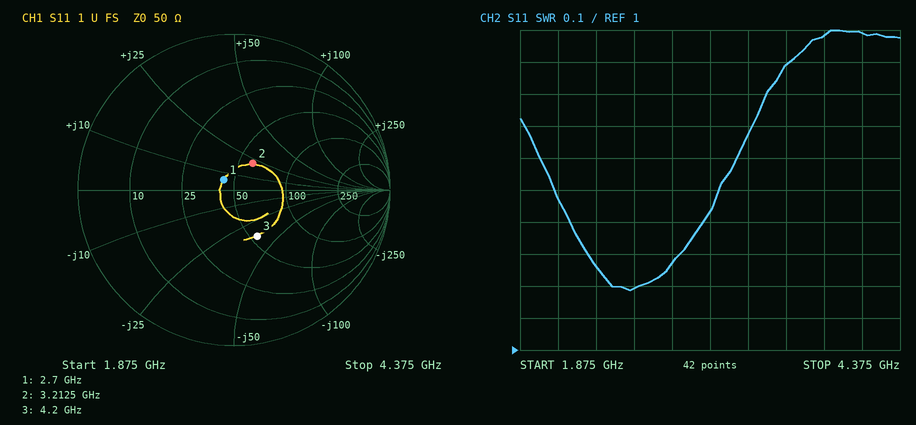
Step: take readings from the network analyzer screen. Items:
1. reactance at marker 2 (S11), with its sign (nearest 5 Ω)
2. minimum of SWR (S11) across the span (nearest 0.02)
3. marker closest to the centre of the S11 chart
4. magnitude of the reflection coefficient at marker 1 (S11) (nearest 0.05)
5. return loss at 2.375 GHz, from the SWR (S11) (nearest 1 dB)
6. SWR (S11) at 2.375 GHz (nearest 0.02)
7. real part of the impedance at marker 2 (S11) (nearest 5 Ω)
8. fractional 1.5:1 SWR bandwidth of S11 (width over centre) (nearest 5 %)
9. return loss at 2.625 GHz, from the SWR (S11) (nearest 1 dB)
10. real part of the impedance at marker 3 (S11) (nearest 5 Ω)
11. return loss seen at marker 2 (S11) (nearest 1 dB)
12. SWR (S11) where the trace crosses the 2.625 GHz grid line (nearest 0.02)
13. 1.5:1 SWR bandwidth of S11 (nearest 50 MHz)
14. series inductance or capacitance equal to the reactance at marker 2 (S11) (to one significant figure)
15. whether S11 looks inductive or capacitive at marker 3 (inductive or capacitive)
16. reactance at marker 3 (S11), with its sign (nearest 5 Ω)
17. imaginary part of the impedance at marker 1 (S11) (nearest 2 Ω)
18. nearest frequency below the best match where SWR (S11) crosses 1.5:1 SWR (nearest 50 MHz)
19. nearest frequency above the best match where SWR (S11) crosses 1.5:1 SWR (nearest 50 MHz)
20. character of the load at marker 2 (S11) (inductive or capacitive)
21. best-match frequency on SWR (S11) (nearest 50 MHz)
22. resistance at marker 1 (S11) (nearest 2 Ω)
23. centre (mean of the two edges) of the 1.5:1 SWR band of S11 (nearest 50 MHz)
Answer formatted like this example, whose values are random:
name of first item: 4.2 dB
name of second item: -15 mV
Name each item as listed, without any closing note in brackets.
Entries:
reactance at marker 2 (S11), with its sign: +20 Ω
minimum of SWR (S11) across the span: 1.18
marker closest to the centre of the S11 chart: marker 1
magnitude of the reflection coefficient at marker 1 (S11): 0.10
return loss at 2.375 GHz, from the SWR (S11): 19 dB
SWR (S11) at 2.375 GHz: 1.26
real part of the impedance at marker 2 (S11): 60 Ω
fractional 1.5:1 SWR bandwidth of S11 (width over centre): 40 %
return loss at 2.625 GHz, from the SWR (S11): 21 dB
real part of the impedance at marker 3 (S11): 55 Ω
return loss seen at marker 2 (S11): 14 dB
SWR (S11) where the trace crosses the 2.625 GHz grid line: 1.20
1.5:1 SWR bandwidth of S11: 1.10 GHz
series inductance or capacitance equal to the reactance at marker 2 (S11): 1 nH
whether S11 looks inductive or capacitive at marker 3: capacitive
reactance at marker 3 (S11), with its sign: -35 Ω
imaginary part of the impedance at marker 1 (S11): +6 Ω
nearest frequency below the best match where SWR (S11) crosses 1.5:1 SWR: 2.10 GHz
nearest frequency above the best match where SWR (S11) crosses 1.5:1 SWR: 3.20 GHz
character of the load at marker 2 (S11): inductive
best-match frequency on SWR (S11): 2.60 GHz
resistance at marker 1 (S11): 44 Ω
centre (mean of the two edges) of the 1.5:1 SWR band of S11: 2.65 GHz
